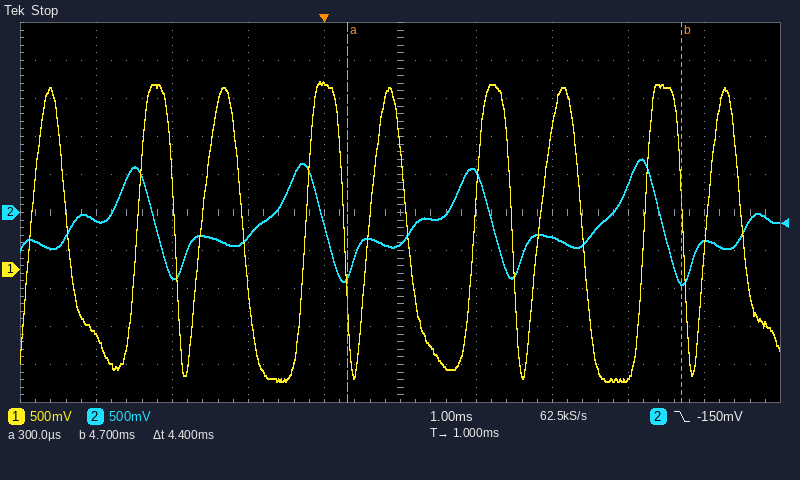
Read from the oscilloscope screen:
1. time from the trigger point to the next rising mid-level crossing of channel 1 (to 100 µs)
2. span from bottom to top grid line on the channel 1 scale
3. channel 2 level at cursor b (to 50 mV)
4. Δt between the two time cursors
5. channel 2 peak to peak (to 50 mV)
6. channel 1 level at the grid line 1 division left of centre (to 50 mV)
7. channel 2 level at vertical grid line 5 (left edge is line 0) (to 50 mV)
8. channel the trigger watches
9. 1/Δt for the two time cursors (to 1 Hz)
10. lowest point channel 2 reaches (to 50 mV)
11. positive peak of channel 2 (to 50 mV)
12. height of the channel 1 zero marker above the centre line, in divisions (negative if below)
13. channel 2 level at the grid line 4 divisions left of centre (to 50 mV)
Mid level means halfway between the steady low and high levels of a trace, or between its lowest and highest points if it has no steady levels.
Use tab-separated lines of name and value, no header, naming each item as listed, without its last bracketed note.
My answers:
time from the trigger point to the next rising mid-level crossing of channel 1	600 µs
span from bottom to top grid line on the channel 1 scale	5 V
channel 2 level at cursor b	-900 mV
Δt between the two time cursors	4.4 ms
channel 2 peak to peak	1.65 V
channel 1 level at the grid line 1 division left of centre	2.45 V
channel 2 level at vertical grid line 5 (left edge is line 0)	-400 mV
channel the trigger watches	channel 2
1/Δt for the two time cursors	227 Hz
lowest point channel 2 reaches	-950 mV
positive peak of channel 2	700 mV
height of the channel 1 zero marker above the centre line, in divisions	-1.5 div
channel 2 level at the grid line 4 divisions left of centre	-100 mV
